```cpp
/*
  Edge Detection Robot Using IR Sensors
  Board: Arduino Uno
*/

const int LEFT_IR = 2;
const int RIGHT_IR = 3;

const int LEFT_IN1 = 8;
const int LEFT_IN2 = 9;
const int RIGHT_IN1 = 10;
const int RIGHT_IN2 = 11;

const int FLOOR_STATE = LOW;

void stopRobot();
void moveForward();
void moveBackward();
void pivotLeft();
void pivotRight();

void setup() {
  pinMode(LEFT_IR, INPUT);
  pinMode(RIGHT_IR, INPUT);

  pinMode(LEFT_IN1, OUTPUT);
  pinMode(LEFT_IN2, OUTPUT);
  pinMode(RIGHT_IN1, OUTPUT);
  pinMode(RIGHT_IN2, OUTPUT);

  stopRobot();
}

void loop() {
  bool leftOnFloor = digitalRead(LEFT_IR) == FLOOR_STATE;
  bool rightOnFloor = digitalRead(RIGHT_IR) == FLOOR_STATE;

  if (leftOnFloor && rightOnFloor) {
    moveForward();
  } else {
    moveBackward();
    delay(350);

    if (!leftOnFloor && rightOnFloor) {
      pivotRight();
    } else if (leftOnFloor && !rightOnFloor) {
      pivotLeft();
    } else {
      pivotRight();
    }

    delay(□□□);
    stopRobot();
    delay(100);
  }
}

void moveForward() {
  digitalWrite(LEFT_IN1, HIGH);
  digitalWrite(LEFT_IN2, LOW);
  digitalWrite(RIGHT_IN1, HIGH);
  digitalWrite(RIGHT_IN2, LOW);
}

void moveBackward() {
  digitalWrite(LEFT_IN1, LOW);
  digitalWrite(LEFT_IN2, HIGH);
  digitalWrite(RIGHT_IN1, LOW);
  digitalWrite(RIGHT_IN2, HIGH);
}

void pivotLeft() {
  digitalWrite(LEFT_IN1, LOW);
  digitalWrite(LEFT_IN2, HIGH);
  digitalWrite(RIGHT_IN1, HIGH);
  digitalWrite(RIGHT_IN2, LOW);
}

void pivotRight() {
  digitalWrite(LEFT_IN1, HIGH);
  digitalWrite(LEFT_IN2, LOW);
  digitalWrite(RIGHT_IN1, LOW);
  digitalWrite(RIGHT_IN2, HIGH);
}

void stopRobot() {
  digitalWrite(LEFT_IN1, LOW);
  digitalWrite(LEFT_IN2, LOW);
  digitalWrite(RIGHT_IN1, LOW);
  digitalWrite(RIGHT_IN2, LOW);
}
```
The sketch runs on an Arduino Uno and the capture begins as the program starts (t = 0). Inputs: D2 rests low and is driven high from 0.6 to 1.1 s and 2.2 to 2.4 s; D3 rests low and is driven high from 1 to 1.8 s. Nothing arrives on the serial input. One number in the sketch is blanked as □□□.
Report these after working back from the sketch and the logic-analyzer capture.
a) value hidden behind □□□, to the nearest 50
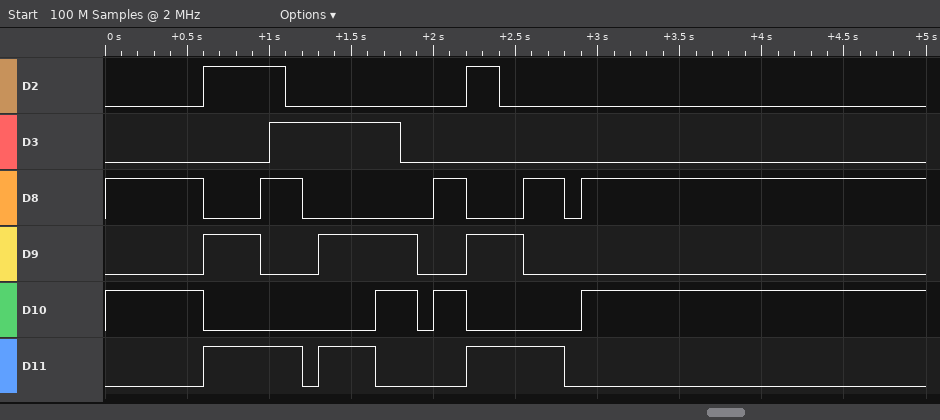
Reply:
250
